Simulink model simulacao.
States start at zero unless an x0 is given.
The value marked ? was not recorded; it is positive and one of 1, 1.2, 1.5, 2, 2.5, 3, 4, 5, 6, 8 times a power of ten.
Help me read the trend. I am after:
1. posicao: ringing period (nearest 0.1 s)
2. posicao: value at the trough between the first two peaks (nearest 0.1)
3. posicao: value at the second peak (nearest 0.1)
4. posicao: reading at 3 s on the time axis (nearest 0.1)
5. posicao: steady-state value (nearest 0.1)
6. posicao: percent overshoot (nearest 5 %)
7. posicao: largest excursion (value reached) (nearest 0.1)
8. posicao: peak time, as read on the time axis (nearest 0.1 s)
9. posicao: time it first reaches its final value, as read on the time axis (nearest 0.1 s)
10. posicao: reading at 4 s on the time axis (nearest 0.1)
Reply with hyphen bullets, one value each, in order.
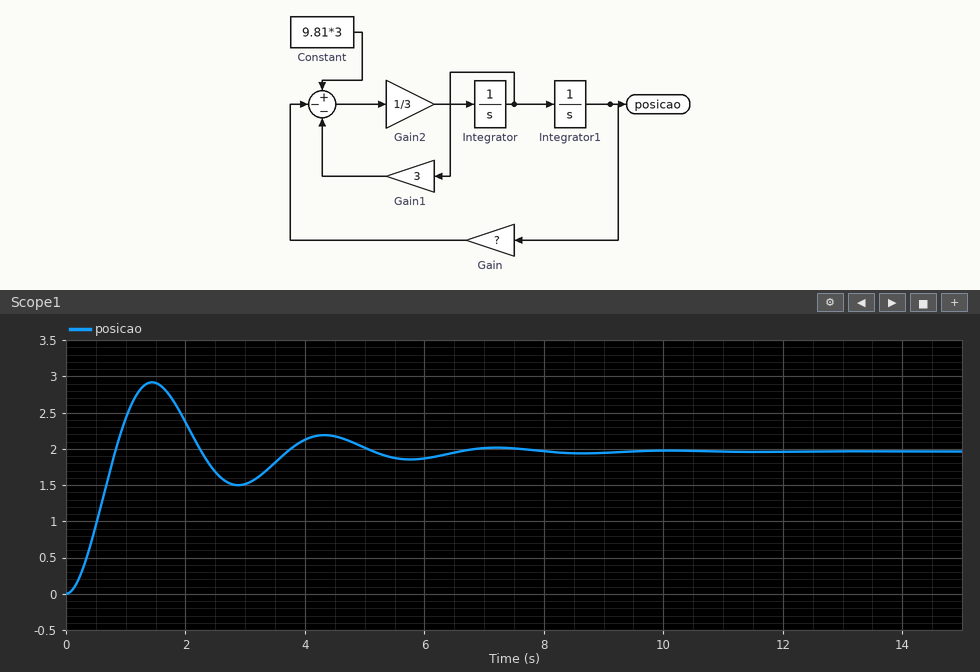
- 2.9 s
- 1.5
- 2.2
- 1.5
- 2.0
- 50 %
- 2.9
- 1.4 s
- 0.8 s
- 2.1
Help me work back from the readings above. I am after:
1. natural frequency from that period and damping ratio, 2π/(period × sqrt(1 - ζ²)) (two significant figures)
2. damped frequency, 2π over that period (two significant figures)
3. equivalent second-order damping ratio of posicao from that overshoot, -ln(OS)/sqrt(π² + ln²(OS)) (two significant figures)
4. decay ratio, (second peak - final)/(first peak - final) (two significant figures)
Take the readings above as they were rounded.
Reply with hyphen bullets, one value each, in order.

- 2.2 rad/s
- 2.2 rad/s
- 0.22
- 0.22
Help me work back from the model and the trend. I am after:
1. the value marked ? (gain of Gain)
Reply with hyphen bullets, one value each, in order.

- 15
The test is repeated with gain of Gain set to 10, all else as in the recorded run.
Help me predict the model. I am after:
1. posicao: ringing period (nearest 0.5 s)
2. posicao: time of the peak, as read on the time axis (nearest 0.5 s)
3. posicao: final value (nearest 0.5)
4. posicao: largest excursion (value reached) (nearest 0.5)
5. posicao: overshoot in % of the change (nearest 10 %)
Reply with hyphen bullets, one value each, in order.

- 3.5 s
- 2.0 s
- 3.0
- 4.0
- 40 %
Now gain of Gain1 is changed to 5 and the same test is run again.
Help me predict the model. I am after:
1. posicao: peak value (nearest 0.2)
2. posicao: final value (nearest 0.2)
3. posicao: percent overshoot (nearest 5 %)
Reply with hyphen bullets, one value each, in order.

- 2.6
- 2.0
- 30 %
